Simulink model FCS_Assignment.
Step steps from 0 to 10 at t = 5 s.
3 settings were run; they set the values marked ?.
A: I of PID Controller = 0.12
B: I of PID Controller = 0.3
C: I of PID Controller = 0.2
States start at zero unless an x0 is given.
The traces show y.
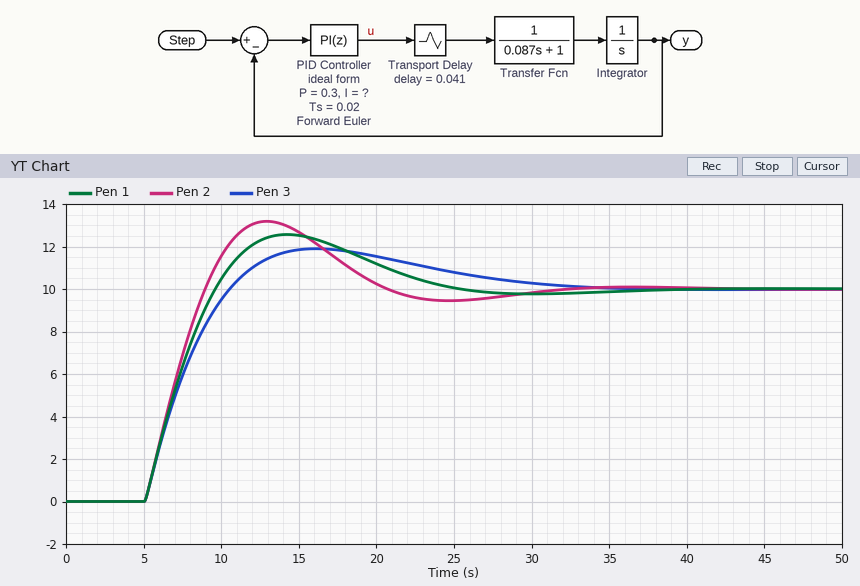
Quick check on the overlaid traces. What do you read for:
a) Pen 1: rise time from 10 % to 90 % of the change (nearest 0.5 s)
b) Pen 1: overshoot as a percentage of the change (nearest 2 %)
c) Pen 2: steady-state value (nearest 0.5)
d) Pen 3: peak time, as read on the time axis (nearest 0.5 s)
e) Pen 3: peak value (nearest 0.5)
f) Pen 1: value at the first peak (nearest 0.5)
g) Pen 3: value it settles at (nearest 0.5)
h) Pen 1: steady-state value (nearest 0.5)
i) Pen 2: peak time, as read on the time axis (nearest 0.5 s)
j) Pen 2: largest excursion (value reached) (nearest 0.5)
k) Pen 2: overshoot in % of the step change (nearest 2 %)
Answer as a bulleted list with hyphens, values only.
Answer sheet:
- 3.5 s
- 26 %
- 10.0
- 16.0 s
- 12.0
- 12.5
- 10.0
- 10.0
- 13.0 s
- 13.0
- 32 %
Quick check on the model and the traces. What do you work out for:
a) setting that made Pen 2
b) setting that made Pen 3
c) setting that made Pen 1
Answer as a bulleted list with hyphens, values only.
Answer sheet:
- B
- A
- C
